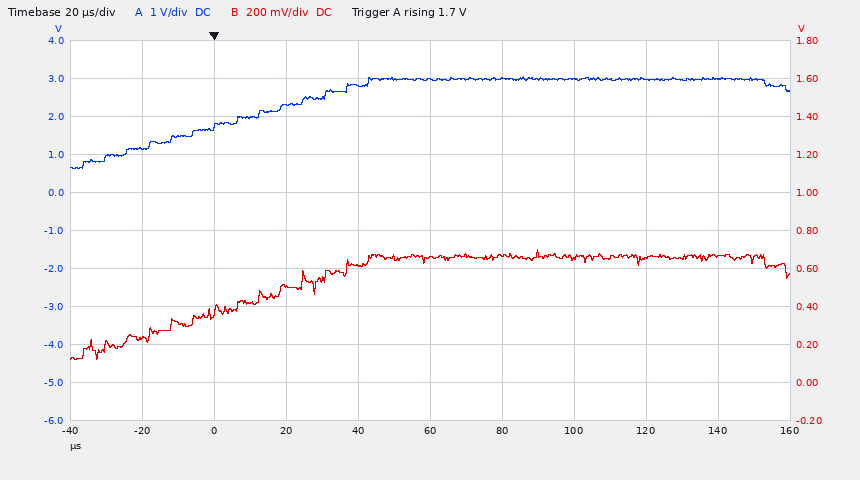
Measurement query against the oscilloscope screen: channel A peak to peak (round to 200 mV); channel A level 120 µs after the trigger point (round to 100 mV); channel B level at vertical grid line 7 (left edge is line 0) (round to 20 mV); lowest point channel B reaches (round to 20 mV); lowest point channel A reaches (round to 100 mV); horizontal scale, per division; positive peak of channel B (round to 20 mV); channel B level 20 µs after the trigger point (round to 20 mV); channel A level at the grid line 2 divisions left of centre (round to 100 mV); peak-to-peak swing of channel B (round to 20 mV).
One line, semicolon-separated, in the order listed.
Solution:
2.4 V; 3.0 V; 660 mV; 120 mV; 600 mV; 20 µs; 700 mV; 500 mV; 2.3 V; 580 mV
